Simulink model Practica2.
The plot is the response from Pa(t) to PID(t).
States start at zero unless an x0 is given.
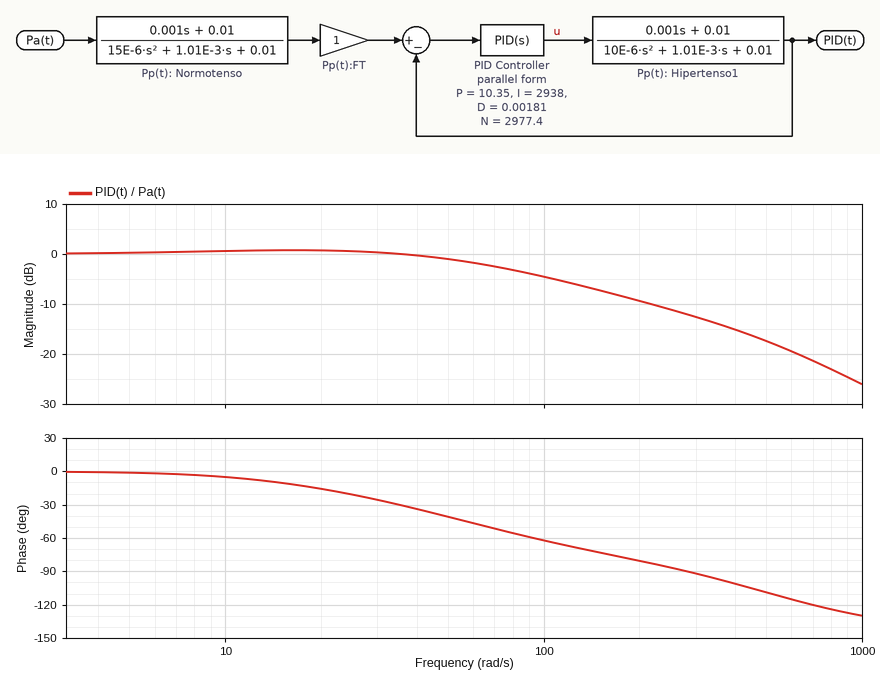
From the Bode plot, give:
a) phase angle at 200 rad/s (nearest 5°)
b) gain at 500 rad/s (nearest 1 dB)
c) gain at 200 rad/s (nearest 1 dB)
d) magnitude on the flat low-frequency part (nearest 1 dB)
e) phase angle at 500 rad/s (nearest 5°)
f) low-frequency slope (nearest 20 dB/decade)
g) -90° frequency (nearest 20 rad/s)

-80°
-17 dB
-9 dB
0 dB
-110°
0 dB/decade
280 rad/s
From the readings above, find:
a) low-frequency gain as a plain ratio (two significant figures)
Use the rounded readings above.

1.0
